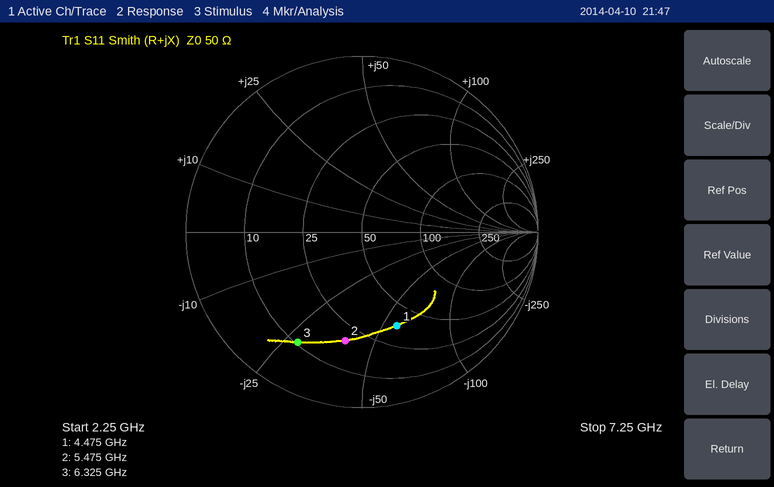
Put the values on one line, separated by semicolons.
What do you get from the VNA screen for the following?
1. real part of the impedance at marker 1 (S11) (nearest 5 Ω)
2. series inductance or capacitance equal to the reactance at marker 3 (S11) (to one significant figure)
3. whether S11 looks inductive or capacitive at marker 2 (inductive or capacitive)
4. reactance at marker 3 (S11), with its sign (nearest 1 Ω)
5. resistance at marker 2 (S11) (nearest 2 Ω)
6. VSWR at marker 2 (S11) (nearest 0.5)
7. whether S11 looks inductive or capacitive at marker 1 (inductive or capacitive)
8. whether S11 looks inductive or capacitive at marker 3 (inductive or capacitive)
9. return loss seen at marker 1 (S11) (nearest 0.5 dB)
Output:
35 Ω; 900 fF; capacitive; -28 Ω; 20 Ω; 4.5; capacitive; capacitive; 5.0 dB
